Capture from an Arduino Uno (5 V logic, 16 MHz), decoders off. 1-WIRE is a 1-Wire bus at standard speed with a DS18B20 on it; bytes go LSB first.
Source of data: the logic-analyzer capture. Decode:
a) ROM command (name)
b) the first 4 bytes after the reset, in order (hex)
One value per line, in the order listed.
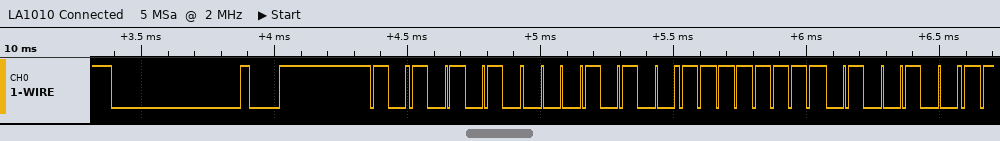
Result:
Match ROM
55 28 FF 92
